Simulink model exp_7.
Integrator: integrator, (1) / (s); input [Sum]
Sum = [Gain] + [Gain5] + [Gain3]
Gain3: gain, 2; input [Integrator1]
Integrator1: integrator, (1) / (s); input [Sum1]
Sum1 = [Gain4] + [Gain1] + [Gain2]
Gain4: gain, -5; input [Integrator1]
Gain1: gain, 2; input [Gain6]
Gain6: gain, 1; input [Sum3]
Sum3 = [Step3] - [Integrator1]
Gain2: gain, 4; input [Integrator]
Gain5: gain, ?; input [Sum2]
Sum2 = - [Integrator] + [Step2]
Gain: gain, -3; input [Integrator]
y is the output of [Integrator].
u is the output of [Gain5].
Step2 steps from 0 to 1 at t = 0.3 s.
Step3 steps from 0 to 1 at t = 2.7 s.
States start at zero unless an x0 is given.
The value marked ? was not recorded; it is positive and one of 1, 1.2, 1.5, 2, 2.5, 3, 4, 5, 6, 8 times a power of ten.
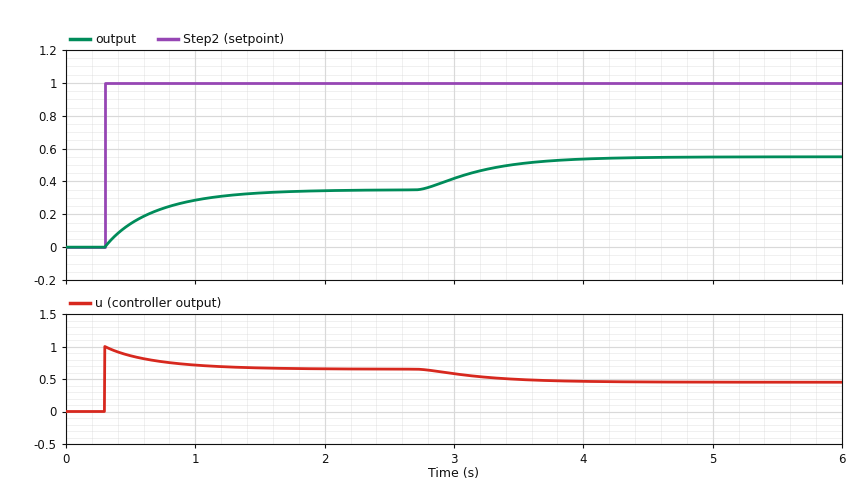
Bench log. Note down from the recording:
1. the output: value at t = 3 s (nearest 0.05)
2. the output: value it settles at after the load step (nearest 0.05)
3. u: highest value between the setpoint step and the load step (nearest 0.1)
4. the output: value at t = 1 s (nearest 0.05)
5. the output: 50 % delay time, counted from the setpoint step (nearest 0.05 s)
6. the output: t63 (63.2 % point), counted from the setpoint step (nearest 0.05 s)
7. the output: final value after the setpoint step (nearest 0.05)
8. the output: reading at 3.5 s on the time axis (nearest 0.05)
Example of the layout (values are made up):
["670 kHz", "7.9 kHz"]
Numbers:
["0.40", "0.55", "1.0", "0.30", "0.25 s", "0.40 s", "0.35", "0.50"]
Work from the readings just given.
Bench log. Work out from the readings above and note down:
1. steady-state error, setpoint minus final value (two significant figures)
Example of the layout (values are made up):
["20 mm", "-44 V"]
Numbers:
["0.65"]
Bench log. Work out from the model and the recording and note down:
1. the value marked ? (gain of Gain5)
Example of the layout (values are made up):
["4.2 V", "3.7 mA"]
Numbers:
["1"]
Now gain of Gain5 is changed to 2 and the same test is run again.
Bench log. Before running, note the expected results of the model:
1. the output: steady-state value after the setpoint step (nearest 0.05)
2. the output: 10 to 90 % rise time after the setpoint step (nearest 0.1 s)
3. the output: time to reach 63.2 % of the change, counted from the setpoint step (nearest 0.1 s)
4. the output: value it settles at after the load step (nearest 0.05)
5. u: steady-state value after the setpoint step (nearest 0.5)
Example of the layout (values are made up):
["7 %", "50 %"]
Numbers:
["0.50", "0.7 s", "0.3 s", "0.65", "1.0"]
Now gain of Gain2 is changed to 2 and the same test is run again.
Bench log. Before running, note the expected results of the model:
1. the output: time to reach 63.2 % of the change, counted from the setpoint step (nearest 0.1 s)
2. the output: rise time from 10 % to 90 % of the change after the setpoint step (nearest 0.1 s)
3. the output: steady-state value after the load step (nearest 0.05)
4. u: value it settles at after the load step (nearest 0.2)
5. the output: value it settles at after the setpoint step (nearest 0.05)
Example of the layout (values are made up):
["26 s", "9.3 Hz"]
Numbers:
["0.3 s", "0.7 s", "0.45", "0.6", "0.30"]
